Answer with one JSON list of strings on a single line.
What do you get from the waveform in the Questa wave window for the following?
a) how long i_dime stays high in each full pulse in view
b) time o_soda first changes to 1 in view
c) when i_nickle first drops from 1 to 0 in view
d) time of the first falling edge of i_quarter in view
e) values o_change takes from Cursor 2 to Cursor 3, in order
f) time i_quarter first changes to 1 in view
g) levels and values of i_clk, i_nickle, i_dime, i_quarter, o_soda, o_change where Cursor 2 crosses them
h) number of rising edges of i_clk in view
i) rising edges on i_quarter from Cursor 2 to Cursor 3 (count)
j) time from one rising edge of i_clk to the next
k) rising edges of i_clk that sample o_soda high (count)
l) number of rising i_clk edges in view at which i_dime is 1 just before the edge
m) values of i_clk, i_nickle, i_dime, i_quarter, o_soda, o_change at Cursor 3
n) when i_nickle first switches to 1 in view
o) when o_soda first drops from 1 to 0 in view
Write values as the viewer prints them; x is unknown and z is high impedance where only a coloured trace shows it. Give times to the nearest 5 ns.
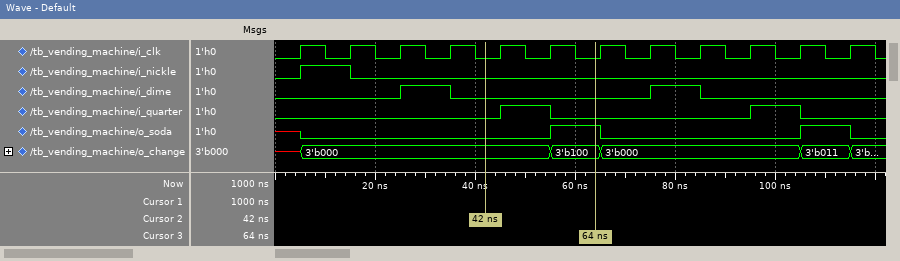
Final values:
["10 ns, 10 ns", "55 ns", "15 ns", "55 ns", "3'b000, 3'b100", "45 ns", "i_clk=0, i_nickle=0, i_dime=0, i_quarter=0, o_soda=0, o_change=3'b000", "12", "1", "10 ns", "2", "2", "i_clk=0, i_nickle=0, i_dime=0, i_quarter=0, o_soda=1, o_change=3'b100", "5 ns", "65 ns"]
